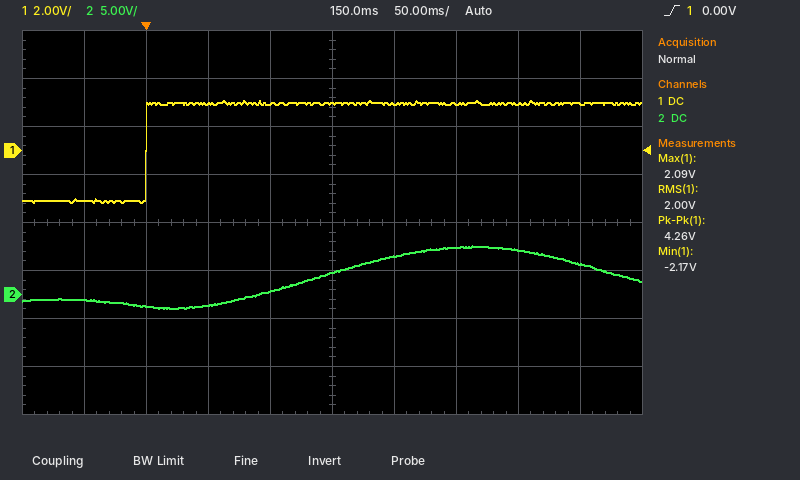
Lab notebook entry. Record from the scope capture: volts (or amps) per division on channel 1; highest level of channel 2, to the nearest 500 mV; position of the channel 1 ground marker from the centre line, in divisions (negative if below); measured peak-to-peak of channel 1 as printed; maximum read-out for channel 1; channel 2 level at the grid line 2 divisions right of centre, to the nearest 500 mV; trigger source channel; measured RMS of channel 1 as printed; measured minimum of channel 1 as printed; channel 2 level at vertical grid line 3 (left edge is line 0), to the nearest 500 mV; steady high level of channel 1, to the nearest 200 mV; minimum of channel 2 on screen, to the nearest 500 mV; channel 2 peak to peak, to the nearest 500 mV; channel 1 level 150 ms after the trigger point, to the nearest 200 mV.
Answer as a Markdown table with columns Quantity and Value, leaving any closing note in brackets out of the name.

| Quantity | Value |
|---|---|
| volts (or amps) per division on channel 1 | 2 V |
| highest level of channel 2, to the nearest 500 mV | 5.0 V |
| position of the channel 1 ground marker from the centre line, in divisions | +1.5 div |
| measured peak-to-peak of channel 1 as printed | 4.26 V |
| maximum read-out for channel 1 | 2.09 V |
| channel 2 level at the grid line 2 divisions right of centre, to the nearest 500 mV | 5.0 V |
| trigger source channel | channel 1 |
| measured RMS of channel 1 as printed | 2.00 V |
| measured minimum of channel 1 as printed | -2.17 V |
| channel 2 level at vertical grid line 3 (left edge is line 0), to the nearest 500 mV | -1.0 V |
| steady high level of channel 1, to the nearest 200 mV | 2.0 V |
| minimum of channel 2 on screen, to the nearest 500 mV | -1.5 V |
| channel 2 peak to peak, to the nearest 500 mV | 6.5 V |
| channel 1 level 150 ms after the trigger point, to the nearest 200 mV | 2.0 V |
